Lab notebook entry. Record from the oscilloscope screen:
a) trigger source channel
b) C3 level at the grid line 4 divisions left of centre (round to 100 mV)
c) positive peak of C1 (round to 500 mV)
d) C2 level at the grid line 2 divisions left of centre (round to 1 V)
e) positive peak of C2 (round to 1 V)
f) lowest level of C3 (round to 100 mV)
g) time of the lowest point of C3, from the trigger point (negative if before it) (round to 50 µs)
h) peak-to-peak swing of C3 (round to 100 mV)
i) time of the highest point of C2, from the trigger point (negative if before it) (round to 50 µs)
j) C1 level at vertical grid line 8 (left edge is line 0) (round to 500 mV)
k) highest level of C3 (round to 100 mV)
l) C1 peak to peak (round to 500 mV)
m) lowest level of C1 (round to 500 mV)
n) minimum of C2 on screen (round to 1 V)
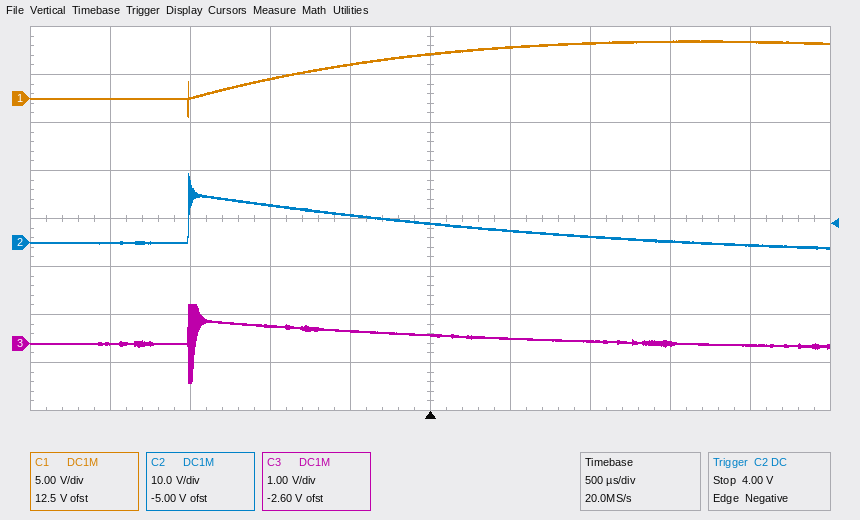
C2
0.0 V
6.0 V
8 V
14 V
-800 mV
-1.50 ms
1.6 V
-1.50 ms
6.0 V
800 mV
8.0 V
-2.0 V
-1 V
